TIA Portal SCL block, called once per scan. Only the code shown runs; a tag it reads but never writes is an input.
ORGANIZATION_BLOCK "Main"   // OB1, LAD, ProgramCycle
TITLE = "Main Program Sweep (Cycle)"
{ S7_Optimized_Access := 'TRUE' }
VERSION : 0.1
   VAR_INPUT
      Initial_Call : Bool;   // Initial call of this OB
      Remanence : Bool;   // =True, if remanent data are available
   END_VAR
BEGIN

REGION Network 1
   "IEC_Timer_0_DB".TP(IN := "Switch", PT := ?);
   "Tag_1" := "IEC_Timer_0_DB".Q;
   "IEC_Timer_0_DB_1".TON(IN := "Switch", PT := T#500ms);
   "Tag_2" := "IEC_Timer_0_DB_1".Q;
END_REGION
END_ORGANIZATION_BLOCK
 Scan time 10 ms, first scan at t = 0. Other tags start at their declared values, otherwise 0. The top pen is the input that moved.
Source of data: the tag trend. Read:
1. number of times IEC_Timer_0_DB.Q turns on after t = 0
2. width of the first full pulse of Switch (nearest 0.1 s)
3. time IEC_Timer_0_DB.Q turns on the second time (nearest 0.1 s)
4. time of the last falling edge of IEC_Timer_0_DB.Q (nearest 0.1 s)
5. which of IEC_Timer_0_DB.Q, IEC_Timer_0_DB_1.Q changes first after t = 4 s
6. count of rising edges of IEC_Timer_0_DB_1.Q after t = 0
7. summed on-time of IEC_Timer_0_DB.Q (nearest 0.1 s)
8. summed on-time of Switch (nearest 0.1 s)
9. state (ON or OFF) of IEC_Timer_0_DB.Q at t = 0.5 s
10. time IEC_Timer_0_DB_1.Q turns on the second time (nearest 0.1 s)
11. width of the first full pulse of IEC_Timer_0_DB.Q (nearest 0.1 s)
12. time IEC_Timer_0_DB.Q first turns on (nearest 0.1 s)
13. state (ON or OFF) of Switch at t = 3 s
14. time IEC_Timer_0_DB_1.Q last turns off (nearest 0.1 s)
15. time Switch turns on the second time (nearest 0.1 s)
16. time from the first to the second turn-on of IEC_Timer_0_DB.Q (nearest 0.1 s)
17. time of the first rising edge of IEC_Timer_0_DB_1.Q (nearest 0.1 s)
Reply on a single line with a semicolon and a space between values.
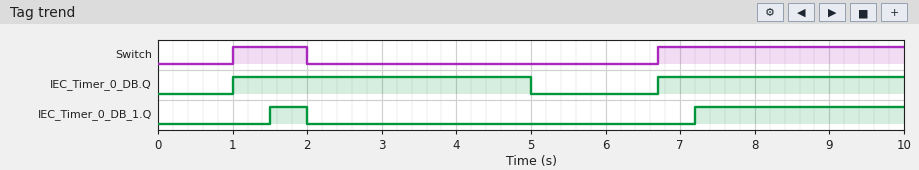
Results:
2; 1.0 s; 6.7 s; 5.0 s; IEC_Timer_0_DB.Q; 2; 7.3 s; 4.3 s; OFF; 7.2 s; 4.0 s; 1.0 s; OFF; 2.0 s; 6.7 s; 5.7 s; 1.5 s
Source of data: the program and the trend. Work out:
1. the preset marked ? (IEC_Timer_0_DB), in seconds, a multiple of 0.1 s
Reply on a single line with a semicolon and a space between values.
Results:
4.0 s
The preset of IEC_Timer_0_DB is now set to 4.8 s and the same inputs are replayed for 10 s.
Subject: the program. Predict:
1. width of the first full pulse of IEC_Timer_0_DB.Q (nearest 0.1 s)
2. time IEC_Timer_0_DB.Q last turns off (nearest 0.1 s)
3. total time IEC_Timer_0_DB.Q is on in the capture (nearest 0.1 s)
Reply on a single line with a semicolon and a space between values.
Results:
4.8 s; 5.8 s; 8.1 s
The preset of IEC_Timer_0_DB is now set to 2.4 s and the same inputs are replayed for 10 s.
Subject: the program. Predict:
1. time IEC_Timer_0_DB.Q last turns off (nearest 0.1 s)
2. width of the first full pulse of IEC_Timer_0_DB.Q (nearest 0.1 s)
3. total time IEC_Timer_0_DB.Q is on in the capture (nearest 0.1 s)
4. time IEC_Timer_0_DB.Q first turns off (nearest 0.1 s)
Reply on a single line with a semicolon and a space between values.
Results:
9.1 s; 2.4 s; 4.8 s; 3.4 s
